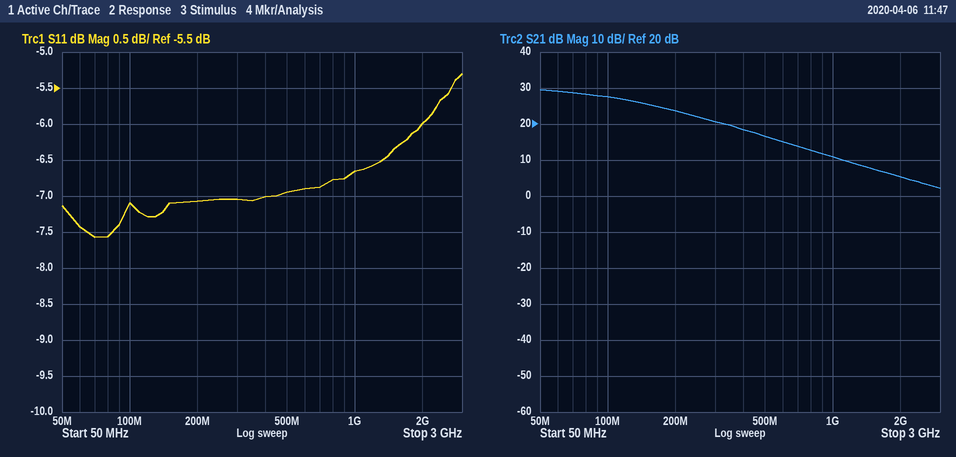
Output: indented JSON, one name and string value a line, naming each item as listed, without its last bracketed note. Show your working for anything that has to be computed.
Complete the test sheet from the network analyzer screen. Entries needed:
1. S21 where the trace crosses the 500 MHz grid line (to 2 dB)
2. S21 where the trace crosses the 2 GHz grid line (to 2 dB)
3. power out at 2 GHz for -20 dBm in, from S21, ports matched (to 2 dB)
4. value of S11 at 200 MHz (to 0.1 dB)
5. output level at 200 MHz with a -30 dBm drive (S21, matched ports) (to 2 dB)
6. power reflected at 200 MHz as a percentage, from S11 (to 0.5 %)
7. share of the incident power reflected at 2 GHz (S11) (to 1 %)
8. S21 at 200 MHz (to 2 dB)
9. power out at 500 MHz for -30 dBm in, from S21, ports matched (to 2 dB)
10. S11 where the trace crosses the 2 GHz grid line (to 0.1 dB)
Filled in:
{
  "S21 where the trace crosses the 500 MHz grid line": "16 dB",
  "S21 where the trace crosses the 2 GHz grid line": "6 dB",
  "power out at 2 GHz for -20 dBm in, from S21, ports matched": "-20 dBm + (6 dB) = -14 dBm",
  "value of S11 at 200 MHz": "-7.1 dB",
  "output level at 200 MHz with a -30 dBm drive (S21, matched ports)": "-30 dBm + (24 dB) = -6 dBm",
  "power reflected at 200 MHz as a percentage, from S11": "10^(-7.1/10) ≈ 19.5 %",
  "share of the incident power reflected at 2 GHz (S11)": "10^(-6/10) ≈ 25 %",
  "S21 at 200 MHz": "24 dB",
  "power out at 500 MHz for -30 dBm in, from S21, ports matched": "-30 dBm + (16 dB) = -14 dBm",
  "S11 where the trace crosses the 2 GHz grid line": "-6.0 dB"
}
